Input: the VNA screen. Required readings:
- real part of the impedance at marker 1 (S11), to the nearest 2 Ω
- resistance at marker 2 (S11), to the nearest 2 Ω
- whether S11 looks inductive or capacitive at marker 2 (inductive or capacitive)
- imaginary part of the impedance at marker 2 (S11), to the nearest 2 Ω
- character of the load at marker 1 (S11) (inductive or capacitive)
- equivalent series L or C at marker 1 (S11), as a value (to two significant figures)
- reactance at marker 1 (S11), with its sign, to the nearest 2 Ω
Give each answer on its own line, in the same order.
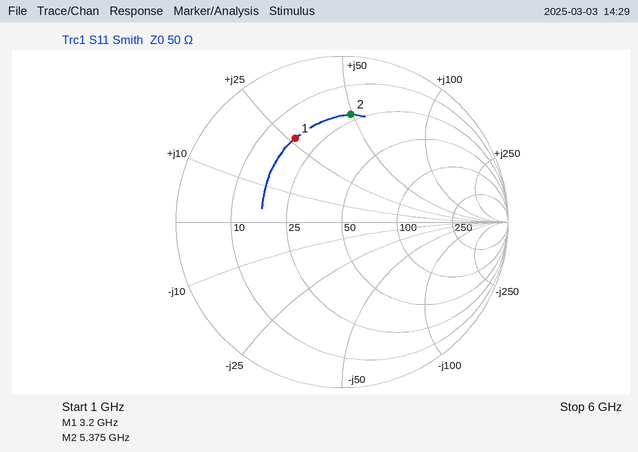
18 Ω
22 Ω
inductive
+50 Ω
inductive
1.3 nH
+26 Ω
